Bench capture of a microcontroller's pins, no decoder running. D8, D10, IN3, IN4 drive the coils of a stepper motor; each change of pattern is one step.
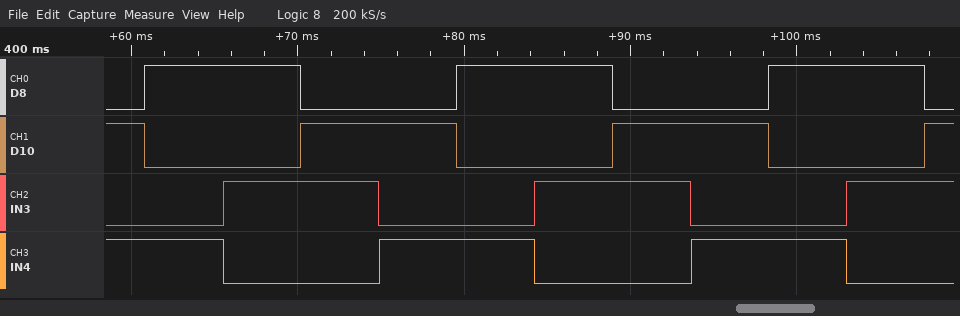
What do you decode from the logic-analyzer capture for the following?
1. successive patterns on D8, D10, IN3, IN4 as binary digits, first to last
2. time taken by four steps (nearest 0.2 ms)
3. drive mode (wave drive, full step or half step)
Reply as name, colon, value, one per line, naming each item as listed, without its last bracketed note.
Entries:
successive patterns on D8, D10, IN3, IN4 as binary digits, first to last: 0101 1001 1010 0110 0101 1001 1010 0110 0101 1001 1010 0110
time taken by four steps: 18.8 ms
drive mode: full step
